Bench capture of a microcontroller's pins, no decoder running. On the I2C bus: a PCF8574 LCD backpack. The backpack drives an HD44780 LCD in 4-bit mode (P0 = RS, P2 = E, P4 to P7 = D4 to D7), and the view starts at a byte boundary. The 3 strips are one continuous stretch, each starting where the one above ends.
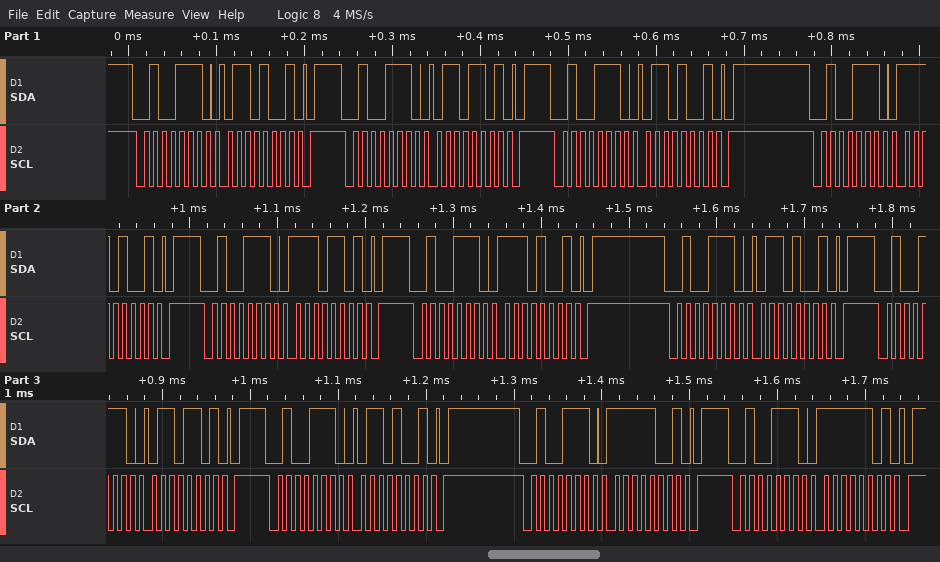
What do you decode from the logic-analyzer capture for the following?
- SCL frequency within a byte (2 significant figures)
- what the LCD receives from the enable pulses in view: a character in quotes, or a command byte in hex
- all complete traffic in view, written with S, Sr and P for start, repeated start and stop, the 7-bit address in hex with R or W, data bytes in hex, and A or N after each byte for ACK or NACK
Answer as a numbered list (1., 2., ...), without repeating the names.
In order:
1. 100 kHz
2. 'n'
3. S 27W A 69 A P S 27W A 6D A P S 27W A 69 A P S 27W A E9 A P S 27W A ED A P S 27W A E9 A P S 27W A 69 A P S 27W A 6D A P S 27W A 69 A P S 27W A F9 A P S 27W A FD A P
